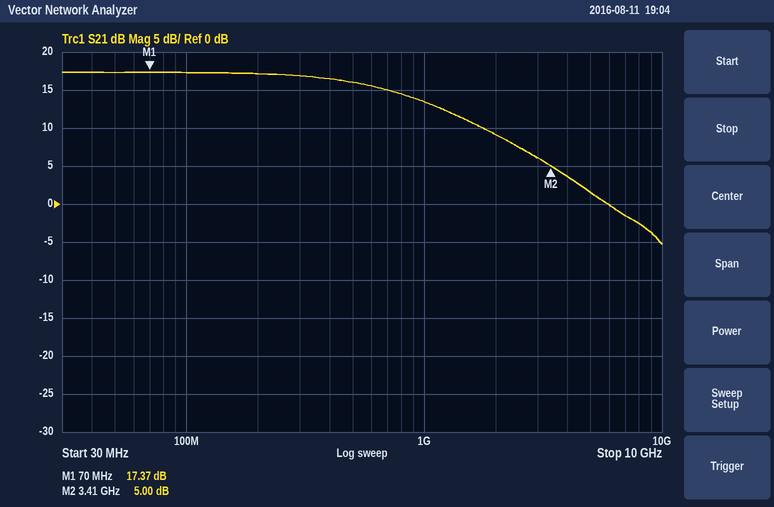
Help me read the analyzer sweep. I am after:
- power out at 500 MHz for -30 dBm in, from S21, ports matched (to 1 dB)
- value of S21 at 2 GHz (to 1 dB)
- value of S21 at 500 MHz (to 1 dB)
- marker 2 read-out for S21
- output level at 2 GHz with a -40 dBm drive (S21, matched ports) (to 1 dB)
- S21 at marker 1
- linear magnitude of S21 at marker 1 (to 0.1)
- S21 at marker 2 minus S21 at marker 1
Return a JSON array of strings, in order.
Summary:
["-14 dBm", "9 dB", "16 dB", "5.00 dB", "-31 dBm", "17.37 dB", "7.4", "-12.37 dB"]
